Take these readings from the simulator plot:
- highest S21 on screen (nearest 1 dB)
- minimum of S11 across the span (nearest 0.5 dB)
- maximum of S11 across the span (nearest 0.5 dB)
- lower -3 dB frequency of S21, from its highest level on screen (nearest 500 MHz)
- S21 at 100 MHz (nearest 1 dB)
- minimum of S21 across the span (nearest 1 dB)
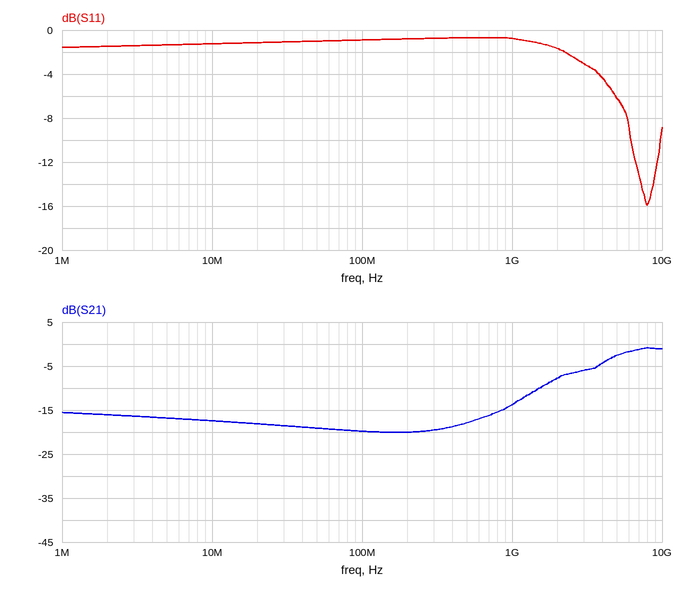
-1 dB
-16.0 dB
-0.5 dB
4.0 GHz
-20 dB
-20 dB
